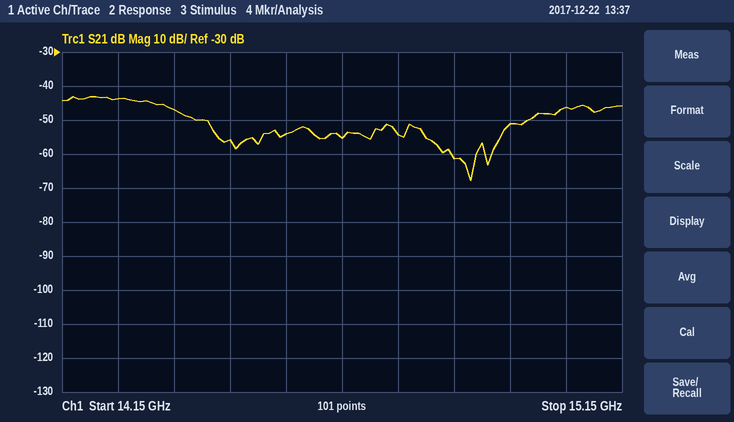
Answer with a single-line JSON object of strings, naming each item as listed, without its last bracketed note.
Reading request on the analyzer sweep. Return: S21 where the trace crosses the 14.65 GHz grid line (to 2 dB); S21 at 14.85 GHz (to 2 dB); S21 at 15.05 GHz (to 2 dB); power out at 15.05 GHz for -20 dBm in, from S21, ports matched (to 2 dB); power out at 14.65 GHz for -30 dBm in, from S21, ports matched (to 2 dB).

{"S21 where the trace crosses the 14.65 GHz grid line": "-56 dB", "S21 at 14.85 GHz": "-62 dB", "S21 at 15.05 GHz": "-46 dB", "power out at 15.05 GHz for -20 dBm in, from S21, ports matched": "-66 dBm", "power out at 14.65 GHz for -30 dBm in, from S21, ports matched": "-86 dBm"}
